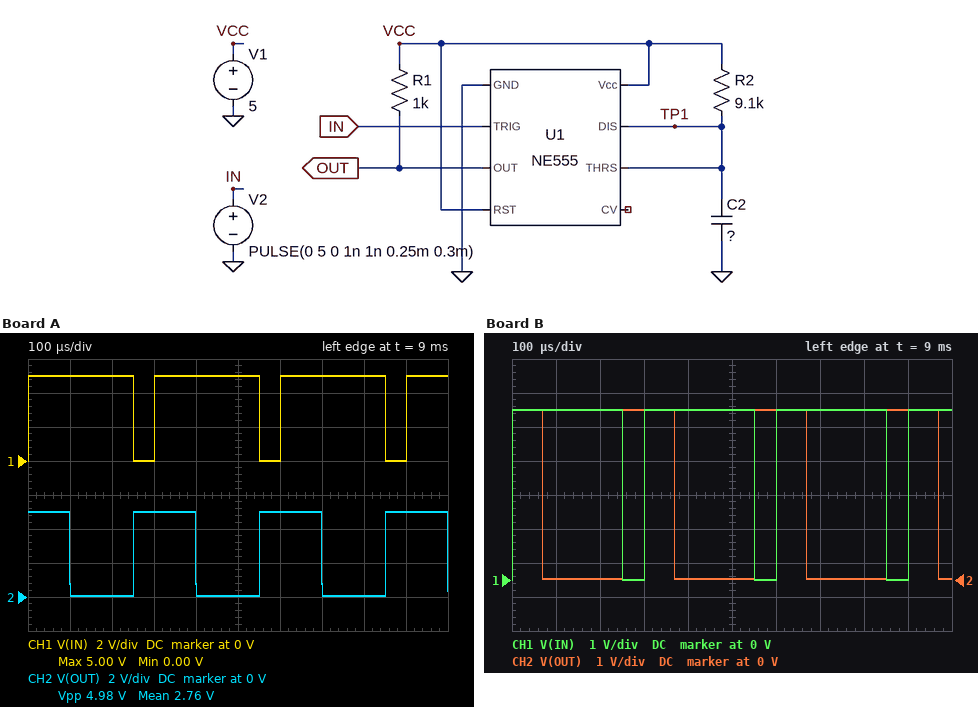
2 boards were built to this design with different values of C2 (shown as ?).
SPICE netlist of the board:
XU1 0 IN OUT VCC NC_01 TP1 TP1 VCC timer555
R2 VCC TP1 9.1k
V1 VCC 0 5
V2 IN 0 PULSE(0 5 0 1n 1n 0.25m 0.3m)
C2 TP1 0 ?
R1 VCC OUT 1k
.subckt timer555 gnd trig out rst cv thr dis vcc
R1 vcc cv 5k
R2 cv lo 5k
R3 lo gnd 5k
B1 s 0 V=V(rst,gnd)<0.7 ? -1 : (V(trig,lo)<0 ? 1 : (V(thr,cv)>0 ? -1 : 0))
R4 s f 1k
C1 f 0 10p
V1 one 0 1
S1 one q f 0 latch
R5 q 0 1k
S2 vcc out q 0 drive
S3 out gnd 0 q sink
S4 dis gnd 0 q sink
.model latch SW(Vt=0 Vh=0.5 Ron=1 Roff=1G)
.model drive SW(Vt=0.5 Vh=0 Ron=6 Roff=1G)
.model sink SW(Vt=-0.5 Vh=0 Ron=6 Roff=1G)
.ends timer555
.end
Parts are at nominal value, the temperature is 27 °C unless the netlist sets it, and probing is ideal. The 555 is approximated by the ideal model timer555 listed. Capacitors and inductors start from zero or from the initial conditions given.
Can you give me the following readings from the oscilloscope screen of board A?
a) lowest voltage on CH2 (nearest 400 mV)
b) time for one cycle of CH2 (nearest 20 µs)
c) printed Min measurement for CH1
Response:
0 V
300 µs
0.00 V
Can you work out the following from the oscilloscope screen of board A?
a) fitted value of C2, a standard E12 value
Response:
15 nF
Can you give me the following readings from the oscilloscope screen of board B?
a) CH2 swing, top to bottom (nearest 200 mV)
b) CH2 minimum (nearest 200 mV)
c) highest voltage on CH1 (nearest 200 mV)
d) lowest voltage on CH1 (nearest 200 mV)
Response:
5.0 V
0 V
5.0 V
0 V
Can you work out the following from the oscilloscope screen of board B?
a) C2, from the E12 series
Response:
12 nF
